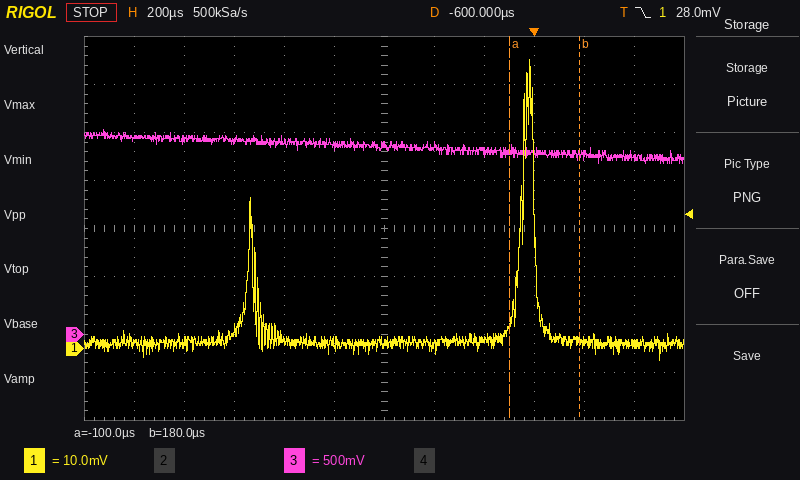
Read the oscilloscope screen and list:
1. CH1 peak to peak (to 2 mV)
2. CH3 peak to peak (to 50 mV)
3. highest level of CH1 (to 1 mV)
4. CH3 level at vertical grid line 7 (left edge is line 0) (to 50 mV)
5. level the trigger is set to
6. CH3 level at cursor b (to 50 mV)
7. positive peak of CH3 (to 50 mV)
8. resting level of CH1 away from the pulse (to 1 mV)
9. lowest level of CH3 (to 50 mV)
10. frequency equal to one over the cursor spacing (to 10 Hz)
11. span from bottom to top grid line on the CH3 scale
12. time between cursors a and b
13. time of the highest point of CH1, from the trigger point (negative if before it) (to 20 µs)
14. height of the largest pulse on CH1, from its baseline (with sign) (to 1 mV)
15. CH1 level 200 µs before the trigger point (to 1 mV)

62 mV
350 mV
60 mV
1.95 V
28.0 mV
1.85 V
2.15 V
1 mV
1.80 V
3.57 kHz
4 V
280 µs
-20 µs
+59 mV
2 mV
